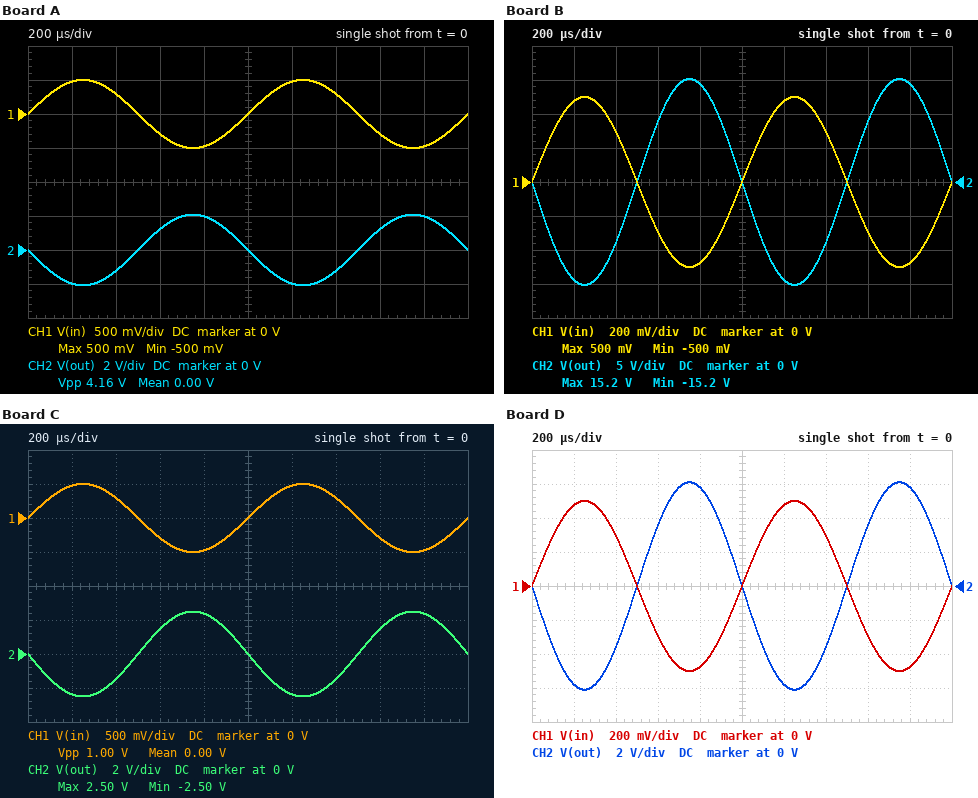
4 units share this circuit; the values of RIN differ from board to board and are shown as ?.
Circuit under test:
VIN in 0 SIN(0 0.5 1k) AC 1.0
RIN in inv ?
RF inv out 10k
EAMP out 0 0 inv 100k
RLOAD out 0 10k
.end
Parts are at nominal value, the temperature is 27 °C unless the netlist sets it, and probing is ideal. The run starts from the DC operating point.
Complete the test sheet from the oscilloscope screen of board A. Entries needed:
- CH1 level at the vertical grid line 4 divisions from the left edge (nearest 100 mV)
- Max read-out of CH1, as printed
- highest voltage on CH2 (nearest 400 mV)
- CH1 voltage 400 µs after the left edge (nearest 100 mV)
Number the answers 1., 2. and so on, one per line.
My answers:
1. -500 mV
2. 500 mV
3. 2.0 V
4. 300 mV
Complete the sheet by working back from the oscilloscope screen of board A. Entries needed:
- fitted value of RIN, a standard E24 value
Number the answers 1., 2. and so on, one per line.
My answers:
1. 2.4 kΩ
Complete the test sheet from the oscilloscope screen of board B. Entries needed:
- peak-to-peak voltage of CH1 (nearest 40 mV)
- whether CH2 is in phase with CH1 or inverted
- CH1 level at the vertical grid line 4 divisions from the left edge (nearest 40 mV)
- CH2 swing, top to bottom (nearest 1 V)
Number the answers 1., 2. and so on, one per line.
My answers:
1. 1.00 V
2. inverted
3. -480 mV
4. 30 V
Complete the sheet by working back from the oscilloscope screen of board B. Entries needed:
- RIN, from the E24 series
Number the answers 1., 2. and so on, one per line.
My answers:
1. 330 Ω
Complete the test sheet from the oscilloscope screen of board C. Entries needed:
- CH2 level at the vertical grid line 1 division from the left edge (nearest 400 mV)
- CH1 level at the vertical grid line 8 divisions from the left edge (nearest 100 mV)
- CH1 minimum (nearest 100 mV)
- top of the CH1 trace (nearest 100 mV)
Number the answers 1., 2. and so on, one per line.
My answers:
1. -2.4 V
2. -300 mV
3. -500 mV
4. 500 mV
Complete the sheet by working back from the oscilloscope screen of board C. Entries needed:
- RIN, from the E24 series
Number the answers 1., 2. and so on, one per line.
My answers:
1. 2 kΩ
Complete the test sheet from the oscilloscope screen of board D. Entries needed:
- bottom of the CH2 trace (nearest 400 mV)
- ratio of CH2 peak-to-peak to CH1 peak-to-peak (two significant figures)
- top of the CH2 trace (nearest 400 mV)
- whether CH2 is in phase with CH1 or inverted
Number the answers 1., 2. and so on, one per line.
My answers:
1. -6.0 V
2. 12
3. 6.0 V
4. inverted
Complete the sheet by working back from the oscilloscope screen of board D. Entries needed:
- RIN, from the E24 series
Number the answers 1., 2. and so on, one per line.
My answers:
1. 820 Ω
